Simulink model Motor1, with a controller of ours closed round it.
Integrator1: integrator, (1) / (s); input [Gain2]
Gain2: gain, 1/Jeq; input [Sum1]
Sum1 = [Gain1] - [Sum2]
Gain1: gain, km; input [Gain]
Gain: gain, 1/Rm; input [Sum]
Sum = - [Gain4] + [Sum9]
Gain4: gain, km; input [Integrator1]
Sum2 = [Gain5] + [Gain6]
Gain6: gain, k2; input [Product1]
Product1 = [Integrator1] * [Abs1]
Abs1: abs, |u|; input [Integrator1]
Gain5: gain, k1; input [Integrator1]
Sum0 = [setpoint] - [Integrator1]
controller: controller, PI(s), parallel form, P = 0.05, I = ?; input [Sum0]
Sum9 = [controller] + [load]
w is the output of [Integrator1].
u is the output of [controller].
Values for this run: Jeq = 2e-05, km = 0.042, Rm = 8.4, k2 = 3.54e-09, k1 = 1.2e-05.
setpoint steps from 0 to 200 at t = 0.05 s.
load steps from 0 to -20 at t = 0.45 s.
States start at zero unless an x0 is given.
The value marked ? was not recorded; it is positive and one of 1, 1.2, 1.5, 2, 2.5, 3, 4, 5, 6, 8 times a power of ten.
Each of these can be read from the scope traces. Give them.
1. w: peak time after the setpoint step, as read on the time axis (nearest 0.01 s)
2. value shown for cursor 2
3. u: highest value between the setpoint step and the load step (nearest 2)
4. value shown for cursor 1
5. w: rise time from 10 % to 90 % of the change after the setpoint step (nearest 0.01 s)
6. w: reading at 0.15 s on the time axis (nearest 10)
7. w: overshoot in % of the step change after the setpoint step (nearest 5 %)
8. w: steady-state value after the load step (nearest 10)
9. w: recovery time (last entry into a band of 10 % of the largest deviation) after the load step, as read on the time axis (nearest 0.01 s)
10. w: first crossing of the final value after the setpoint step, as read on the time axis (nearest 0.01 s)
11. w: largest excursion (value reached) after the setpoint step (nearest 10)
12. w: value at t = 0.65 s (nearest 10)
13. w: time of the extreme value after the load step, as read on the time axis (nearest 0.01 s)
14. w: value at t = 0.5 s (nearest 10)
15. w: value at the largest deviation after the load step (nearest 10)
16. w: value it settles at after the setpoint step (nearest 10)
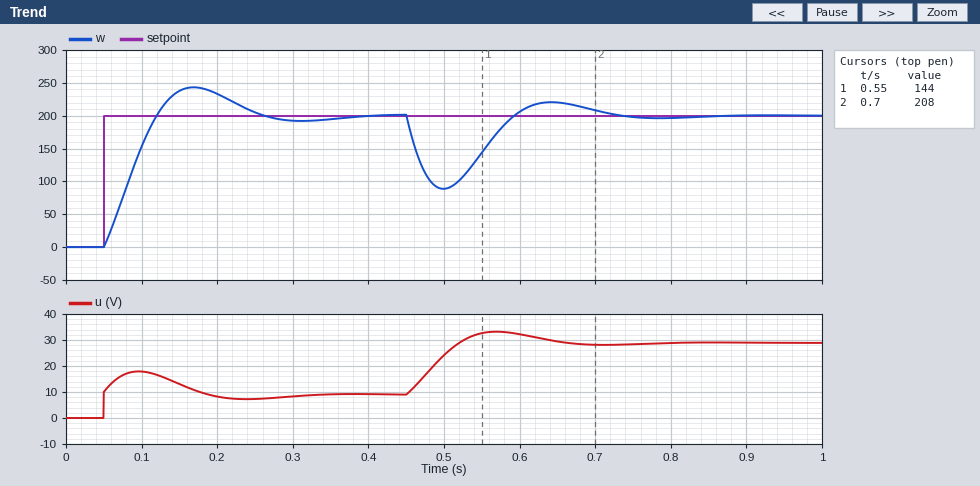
0.17 s
208
18
144
0.05 s
240
20 %
200
0.69 s
0.12 s
240
220
0.50 s
90
90
200
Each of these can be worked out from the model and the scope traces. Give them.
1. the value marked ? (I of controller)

2.5
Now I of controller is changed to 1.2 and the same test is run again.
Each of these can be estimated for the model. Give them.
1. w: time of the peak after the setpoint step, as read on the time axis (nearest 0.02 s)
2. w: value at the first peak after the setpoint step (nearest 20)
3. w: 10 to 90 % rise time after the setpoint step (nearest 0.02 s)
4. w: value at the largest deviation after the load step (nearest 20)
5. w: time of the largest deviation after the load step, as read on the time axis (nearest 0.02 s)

0.24 s
220
0.08 s
60
0.52 s
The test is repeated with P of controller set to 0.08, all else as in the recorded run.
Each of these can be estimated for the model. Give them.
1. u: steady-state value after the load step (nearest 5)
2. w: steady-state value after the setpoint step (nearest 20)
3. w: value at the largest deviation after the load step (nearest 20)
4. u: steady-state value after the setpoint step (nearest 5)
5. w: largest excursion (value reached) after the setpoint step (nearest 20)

30
200
100
10
220
